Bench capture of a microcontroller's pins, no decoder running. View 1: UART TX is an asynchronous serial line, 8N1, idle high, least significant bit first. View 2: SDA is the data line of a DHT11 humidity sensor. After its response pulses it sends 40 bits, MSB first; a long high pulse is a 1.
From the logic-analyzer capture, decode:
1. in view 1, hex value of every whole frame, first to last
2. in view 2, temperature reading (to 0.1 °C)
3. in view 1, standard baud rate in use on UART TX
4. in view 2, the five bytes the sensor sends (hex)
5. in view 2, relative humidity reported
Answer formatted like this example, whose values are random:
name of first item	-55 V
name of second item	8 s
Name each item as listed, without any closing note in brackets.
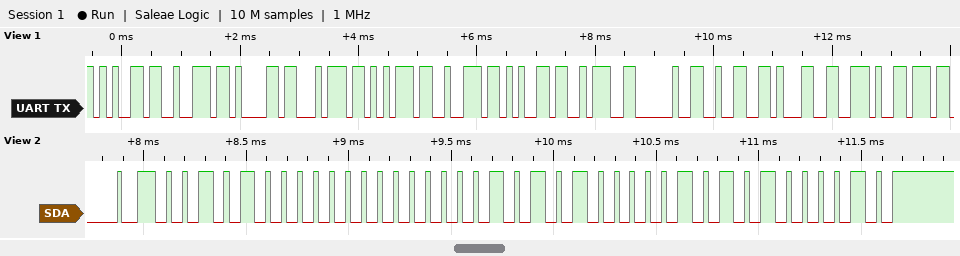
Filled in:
in view 1, hex value of every whole frame, first to last	0x65 0x72 0x61 0x74 0x75 0x72 0x65 0x3A 0x20 0x32 0x31 0x2E
in view 2, temperature reading	21.5 °C
in view 1, standard baud rate in use on UART TX	9600 baud
in view 2, the five bytes the sensor sends	28 00 15 05 42
in view 2, relative humidity reported	40 %
